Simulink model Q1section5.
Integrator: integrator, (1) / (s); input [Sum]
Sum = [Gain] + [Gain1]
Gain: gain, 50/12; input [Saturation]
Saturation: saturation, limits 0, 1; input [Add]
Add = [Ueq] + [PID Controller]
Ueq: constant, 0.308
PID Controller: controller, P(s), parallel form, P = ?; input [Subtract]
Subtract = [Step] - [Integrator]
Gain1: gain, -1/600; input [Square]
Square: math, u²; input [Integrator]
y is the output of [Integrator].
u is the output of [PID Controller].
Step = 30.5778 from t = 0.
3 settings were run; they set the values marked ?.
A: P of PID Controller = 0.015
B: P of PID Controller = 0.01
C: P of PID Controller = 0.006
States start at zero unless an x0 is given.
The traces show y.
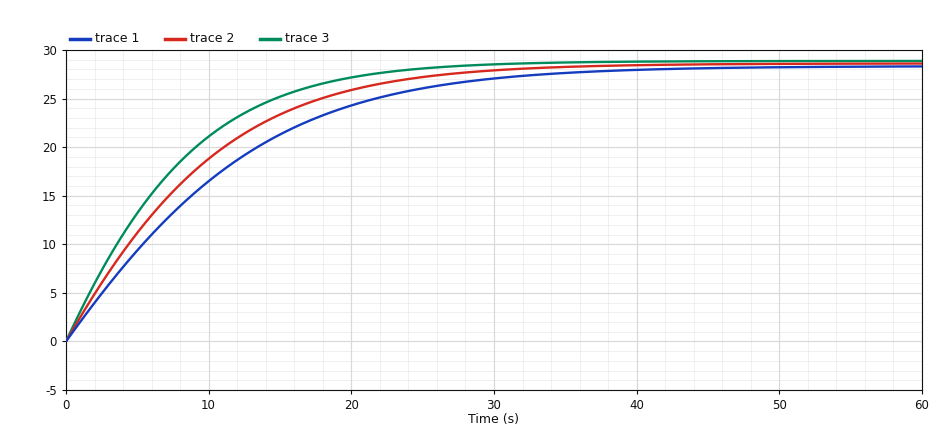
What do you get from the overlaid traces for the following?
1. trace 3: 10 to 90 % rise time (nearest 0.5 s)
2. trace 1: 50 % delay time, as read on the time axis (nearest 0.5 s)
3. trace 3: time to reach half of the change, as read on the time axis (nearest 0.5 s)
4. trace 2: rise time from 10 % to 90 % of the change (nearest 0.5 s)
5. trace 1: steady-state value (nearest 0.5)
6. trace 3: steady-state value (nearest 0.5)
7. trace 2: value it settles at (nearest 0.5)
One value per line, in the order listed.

15.5 s
8.0 s
5.5 s
18.5 s
28.5
29.0
28.5
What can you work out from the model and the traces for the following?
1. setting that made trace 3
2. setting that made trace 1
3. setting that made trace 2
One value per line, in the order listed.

A
C
B
